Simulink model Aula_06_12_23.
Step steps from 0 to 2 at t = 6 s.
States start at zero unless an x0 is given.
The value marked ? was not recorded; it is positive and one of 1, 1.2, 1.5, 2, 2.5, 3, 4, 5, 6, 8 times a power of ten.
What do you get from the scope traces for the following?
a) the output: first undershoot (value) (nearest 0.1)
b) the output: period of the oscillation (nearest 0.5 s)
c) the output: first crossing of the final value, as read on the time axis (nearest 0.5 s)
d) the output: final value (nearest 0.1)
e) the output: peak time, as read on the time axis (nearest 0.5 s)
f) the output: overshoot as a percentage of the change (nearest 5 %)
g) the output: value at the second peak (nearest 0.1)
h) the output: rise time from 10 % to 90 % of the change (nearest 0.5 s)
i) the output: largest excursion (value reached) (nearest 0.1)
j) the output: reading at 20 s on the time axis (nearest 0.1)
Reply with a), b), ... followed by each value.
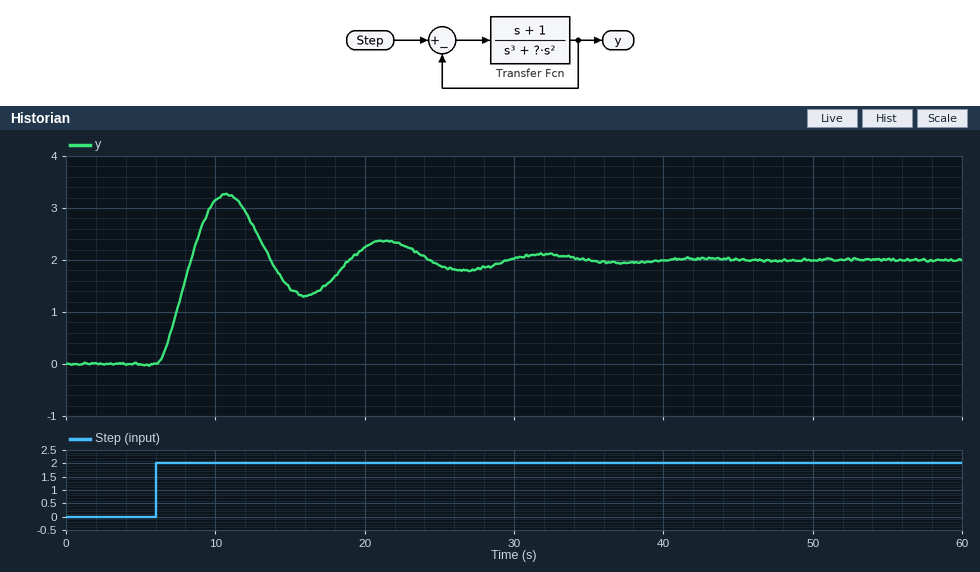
a) 1.3
b) 10.5 s
c) 8.5 s
d) 2.0
e) 10.5 s
f) 65 %
g) 2.4
h) 1.5 s
i) 3.3
j) 2.2
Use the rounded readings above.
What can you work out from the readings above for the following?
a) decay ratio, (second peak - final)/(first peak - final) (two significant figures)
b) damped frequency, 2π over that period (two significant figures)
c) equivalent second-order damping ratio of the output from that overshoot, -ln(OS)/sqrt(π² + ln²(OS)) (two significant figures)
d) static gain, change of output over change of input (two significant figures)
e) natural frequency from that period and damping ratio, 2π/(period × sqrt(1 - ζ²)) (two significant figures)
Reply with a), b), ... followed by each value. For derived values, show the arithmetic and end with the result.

a) (2.4 - 2) / (3.3 - 2) = 0.31
b) 2π / 10.5 = 0.60 rad/s
c) ln(0.65) = -0.431; 0.431 / sqrt(9.870 + 0.186) = 0.14
d) (2 - 0) / (2 - 0) = 1.0
e) 2π / (10.5 × sqrt(1 - 0.14²)) = 0.60 rad/s
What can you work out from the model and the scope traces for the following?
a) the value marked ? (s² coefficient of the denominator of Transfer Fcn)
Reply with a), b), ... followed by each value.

a) 3
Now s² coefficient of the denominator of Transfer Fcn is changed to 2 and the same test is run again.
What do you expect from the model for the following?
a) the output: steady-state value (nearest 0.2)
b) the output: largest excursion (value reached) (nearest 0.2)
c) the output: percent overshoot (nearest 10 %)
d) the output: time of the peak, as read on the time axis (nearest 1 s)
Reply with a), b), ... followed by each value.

a) 2.0
b) 3.4
c) 70 %
d) 10 s
